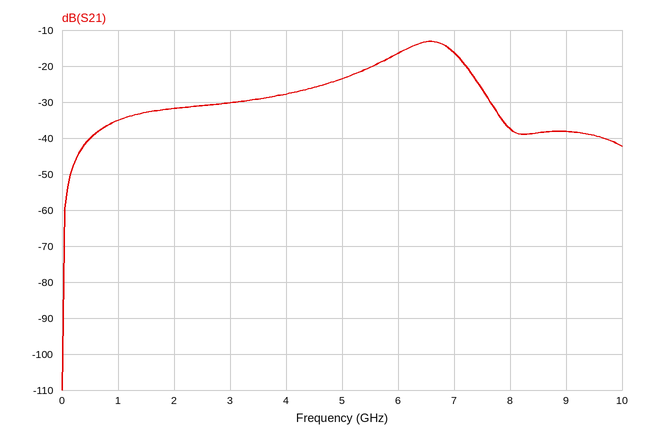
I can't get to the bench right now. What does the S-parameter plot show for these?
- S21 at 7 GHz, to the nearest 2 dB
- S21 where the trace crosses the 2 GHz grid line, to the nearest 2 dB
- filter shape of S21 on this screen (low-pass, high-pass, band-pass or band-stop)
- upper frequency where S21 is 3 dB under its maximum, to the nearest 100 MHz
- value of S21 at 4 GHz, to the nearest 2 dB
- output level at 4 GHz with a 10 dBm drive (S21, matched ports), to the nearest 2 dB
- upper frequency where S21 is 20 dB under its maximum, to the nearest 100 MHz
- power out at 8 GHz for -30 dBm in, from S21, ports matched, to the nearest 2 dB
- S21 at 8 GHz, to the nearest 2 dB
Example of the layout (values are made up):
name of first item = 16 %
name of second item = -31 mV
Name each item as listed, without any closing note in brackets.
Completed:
S21 at 7 GHz, to the nearest 2 dB = -16 dB
S21 where the trace crosses the 2 GHz grid line, to the nearest 2 dB = -32 dB
filter shape of S21 on this screen = band-pass
upper frequency where S21 is 3 dB under its maximum, to the nearest 100 MHz = 7.0 GHz
value of S21 at 4 GHz, to the nearest 2 dB = -28 dB
output level at 4 GHz with a 10 dBm drive (S21, matched ports), to the nearest 2 dB = -18 dBm
upper frequency where S21 is 20 dB under its maximum, to the nearest 100 MHz = 7.8 GHz
power out at 8 GHz for -30 dBm in, from S21, ports matched, to the nearest 2 dB = -68 dBm
S21 at 8 GHz, to the nearest 2 dB = -38 dB
